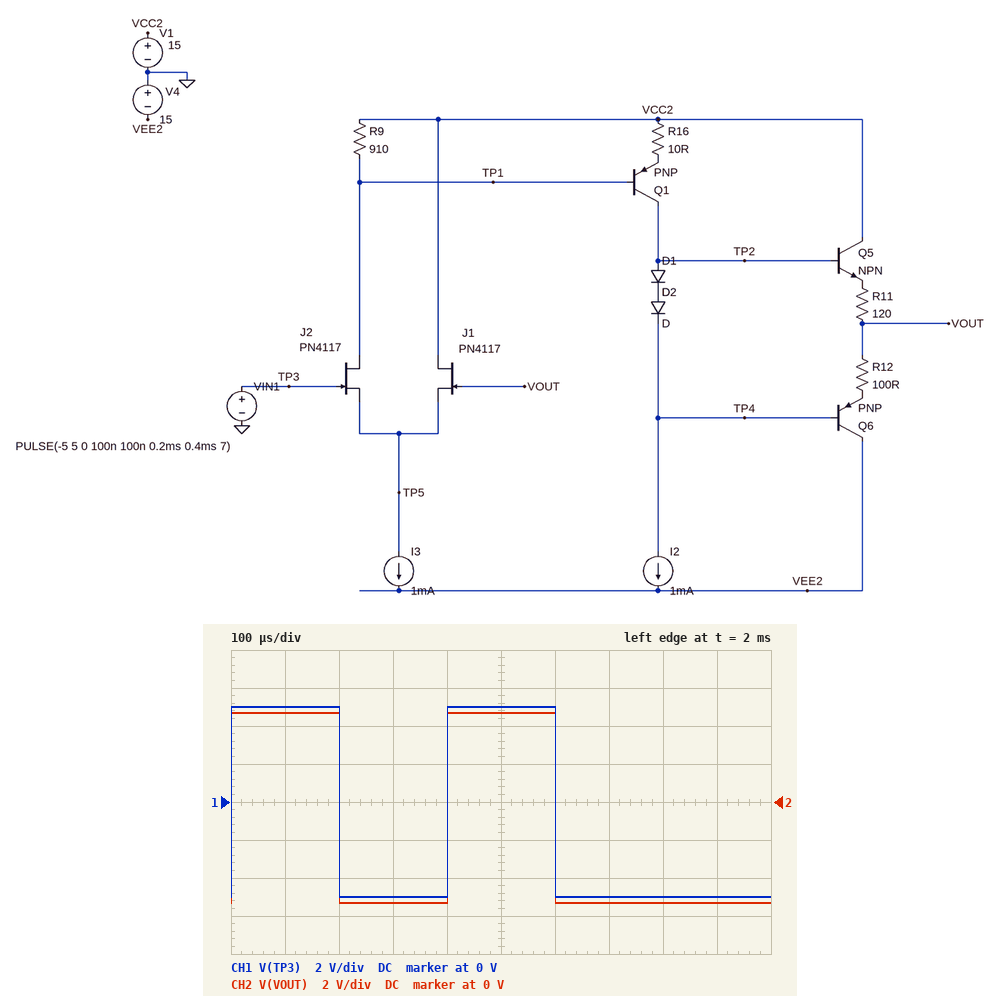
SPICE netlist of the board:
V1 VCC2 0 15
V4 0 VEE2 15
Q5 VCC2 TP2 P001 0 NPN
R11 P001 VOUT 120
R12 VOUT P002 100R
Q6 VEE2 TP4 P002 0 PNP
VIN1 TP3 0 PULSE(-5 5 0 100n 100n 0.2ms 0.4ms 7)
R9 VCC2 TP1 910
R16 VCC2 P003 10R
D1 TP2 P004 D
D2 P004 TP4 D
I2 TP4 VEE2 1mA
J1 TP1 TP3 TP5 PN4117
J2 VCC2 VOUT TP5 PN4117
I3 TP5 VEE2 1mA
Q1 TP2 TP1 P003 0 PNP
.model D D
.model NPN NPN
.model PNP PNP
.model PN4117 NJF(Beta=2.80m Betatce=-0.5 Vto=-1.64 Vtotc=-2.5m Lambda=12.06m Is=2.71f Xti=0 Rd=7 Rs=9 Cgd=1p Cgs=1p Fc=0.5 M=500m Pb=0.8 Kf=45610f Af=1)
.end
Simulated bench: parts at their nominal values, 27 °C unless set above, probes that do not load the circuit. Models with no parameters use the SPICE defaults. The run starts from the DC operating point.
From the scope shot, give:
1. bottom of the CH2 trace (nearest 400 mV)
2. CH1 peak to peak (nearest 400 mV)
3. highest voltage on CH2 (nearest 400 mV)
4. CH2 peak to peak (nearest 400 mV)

-5.2 V
10.0 V
4.8 V
10.0 V
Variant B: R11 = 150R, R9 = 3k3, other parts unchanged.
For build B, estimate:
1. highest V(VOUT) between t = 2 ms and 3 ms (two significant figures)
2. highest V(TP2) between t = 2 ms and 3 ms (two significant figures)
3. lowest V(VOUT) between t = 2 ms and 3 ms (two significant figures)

5.2 V
5.9 V
-4.8 V
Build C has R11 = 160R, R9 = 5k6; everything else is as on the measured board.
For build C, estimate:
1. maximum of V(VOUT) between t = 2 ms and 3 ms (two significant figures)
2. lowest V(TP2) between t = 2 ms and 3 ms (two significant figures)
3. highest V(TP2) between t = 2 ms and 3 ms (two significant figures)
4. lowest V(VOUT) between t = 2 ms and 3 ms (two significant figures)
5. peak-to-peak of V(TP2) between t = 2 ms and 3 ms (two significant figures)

5.3 V
-4.1 V
6.0 V
-4.7 V
10 V
